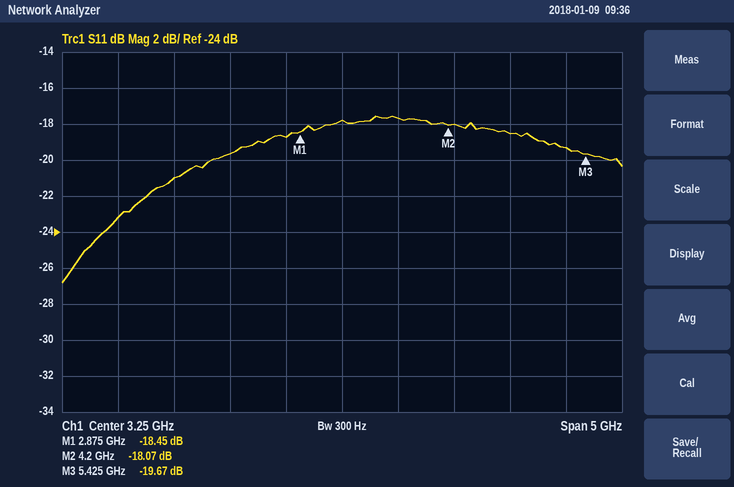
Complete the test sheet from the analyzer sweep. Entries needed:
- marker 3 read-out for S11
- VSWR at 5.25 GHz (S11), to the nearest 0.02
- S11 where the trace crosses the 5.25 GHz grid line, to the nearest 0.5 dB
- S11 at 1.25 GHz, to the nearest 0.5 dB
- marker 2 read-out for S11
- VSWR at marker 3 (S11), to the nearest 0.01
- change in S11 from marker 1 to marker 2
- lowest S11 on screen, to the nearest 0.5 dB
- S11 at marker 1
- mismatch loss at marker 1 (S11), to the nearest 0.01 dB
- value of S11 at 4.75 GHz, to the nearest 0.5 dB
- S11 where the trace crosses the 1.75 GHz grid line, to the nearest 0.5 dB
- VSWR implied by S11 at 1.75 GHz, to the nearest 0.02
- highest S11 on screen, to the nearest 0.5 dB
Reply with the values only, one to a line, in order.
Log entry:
-19.67 dB
1.24
-19.5 dB
-23.0 dB
-18.07 dB
1.23
0.38 dB
-27.0 dB
-18.45 dB
0.06 dB
-18.5 dB
-21.0 dB
1.20
-17.5 dB
